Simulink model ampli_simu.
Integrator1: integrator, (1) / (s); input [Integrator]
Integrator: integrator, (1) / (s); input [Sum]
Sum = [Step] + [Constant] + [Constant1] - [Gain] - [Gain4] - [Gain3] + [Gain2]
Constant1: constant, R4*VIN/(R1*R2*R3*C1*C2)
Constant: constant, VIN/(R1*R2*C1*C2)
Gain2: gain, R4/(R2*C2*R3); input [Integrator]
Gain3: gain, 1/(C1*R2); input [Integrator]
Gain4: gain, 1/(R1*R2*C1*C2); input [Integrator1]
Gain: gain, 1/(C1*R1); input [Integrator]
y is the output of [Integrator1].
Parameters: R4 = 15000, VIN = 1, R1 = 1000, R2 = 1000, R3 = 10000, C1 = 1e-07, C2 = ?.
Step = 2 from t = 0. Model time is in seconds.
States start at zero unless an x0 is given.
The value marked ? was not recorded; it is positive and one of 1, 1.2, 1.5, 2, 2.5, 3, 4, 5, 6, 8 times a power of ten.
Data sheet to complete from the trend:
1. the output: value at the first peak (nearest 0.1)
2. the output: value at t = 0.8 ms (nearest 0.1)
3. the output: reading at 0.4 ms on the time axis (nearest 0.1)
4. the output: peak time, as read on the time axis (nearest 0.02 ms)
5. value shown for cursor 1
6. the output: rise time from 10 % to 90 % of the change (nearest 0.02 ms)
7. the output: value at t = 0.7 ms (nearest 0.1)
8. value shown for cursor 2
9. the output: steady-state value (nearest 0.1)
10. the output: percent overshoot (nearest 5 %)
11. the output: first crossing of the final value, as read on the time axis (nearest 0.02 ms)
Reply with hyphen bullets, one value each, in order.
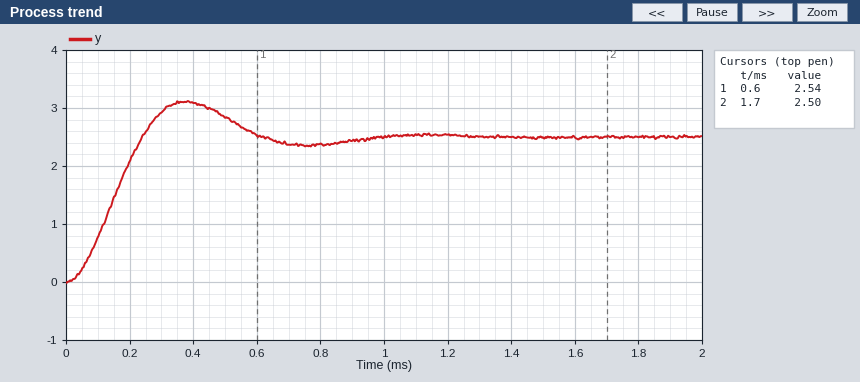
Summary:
- 3.1
- 2.4
- 3.1
- 0.38 ms
- 2.54
- 0.16 ms
- 2.4
- 2.50
- 2.5
- 25 %
- 0.24 ms
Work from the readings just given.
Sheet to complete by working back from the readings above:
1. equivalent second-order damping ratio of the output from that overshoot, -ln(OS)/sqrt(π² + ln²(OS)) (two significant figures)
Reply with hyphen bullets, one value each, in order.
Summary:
- 0.40
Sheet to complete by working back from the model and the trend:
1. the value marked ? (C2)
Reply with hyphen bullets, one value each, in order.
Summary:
- 1.2e-07
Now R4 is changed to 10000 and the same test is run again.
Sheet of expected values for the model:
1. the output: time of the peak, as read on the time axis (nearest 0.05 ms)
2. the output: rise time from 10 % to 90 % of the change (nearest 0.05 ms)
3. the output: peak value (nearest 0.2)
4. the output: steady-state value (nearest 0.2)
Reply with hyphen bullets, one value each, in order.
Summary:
- 0.45 ms
- 0.20 ms
- 2.2
- 2.0
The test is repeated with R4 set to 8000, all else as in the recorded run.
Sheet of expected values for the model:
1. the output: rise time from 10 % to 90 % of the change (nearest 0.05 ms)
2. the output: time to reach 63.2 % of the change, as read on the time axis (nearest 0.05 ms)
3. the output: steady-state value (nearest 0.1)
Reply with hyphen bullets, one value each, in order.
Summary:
- 0.25 ms
- 0.20 ms
- 1.8
